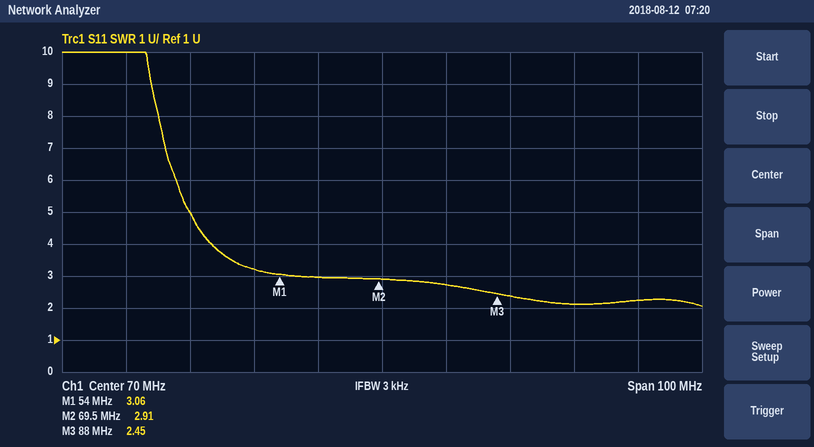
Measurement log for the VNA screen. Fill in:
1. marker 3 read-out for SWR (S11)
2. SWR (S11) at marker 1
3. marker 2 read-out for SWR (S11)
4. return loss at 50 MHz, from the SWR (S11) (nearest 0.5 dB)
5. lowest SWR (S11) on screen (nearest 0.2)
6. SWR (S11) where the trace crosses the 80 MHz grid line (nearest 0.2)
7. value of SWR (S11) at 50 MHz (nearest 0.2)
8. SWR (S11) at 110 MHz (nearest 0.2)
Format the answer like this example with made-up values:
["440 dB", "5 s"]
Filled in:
["2.45", "3.06", "2.91", "5.5 dB", "2.0", "2.8", "3.2", "2.2"]
